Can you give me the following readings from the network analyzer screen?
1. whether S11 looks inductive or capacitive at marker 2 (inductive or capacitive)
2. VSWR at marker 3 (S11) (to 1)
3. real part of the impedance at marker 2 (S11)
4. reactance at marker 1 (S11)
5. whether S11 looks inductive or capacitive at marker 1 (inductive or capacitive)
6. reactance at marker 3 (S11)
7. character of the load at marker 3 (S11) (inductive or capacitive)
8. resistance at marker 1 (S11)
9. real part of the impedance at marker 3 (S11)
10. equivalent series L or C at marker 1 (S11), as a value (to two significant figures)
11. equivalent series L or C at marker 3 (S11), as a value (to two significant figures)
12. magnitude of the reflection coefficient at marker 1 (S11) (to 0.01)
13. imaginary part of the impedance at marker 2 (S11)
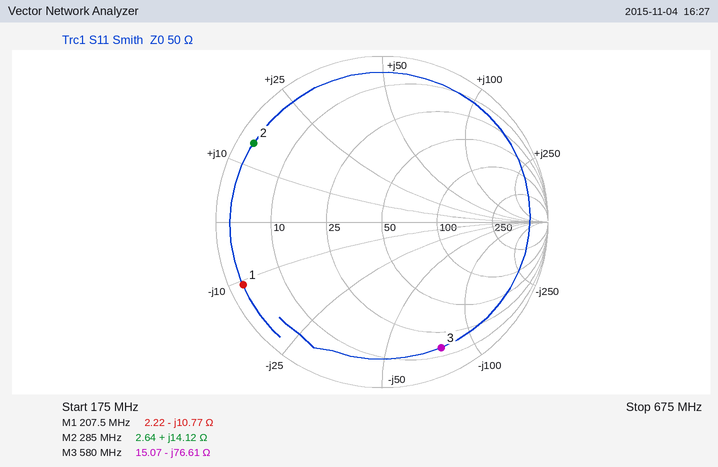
inductive
11
2.64 Ω
-10.77 Ω
capacitive
-76.61 Ω
capacitive
2.22 Ω
15.07 Ω
71 pF
3.6 pF
0.92
+14.12 Ω
